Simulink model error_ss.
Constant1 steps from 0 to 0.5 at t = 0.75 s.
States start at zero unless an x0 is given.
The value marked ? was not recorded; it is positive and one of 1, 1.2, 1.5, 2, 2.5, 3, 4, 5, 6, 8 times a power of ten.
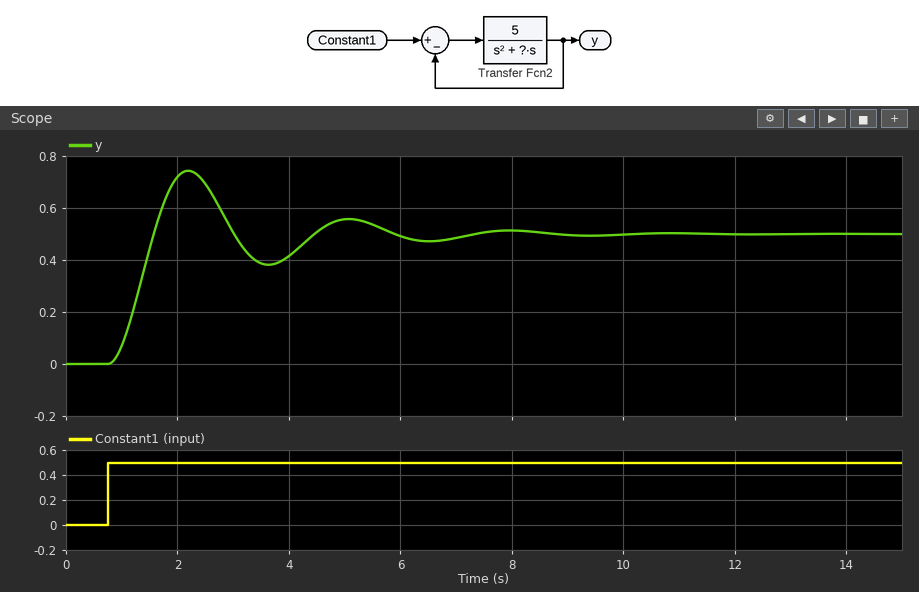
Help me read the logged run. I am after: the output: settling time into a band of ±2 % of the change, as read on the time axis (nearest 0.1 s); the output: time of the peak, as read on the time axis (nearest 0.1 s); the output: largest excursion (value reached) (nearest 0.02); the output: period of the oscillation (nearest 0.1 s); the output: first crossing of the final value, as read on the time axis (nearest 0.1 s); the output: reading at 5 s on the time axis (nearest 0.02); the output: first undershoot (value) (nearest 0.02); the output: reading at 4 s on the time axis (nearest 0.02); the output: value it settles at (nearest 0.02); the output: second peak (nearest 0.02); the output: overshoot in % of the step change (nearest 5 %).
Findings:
8.3 s
2.2 s
0.74
2.9 s
1.6 s
0.56
0.38
0.42
0.50
0.56
50 %
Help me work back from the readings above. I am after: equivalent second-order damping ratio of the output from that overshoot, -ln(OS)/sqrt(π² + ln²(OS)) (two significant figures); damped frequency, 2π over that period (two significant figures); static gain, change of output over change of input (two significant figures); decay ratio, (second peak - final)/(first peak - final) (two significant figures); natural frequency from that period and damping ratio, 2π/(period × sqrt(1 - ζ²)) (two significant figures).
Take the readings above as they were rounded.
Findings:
0.22
2.2 rad/s
1.0
0.25
2.2 rad/s
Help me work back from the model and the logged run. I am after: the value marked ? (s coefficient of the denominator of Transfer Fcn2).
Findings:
1
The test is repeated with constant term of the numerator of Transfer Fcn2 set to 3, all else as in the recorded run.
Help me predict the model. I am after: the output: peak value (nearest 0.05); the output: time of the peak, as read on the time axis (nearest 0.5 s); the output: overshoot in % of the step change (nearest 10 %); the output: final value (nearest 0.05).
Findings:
0.70
2.5 s
40 %
0.50
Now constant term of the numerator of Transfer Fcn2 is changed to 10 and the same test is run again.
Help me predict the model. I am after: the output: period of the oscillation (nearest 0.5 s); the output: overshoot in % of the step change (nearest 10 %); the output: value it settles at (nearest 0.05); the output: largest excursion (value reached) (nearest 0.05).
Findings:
2.0 s
60 %
0.50
0.80
